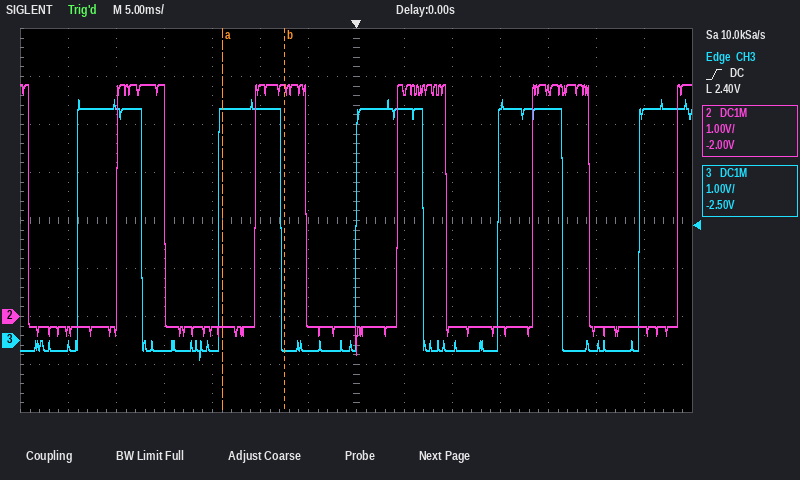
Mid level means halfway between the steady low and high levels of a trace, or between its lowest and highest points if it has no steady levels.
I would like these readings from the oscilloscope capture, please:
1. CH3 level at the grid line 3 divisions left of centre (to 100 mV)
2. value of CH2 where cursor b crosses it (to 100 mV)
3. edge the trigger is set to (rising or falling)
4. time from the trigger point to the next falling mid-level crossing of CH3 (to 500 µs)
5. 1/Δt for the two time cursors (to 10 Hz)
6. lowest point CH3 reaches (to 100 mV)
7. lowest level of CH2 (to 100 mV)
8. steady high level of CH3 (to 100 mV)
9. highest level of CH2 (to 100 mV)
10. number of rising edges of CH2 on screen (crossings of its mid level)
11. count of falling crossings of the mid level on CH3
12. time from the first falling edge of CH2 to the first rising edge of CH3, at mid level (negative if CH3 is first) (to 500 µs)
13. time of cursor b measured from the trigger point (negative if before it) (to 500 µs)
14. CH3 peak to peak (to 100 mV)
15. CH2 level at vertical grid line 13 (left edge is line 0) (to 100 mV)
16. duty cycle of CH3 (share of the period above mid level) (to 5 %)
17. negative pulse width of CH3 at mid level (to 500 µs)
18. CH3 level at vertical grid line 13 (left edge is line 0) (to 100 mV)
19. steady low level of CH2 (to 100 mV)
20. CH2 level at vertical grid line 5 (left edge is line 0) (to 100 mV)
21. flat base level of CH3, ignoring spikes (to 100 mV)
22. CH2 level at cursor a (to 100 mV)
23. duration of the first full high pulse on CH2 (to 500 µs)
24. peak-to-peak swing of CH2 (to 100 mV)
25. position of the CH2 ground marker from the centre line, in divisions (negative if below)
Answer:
-200 mV
4.7 V
rising
7.0 ms
150 Hz
-400 mV
-800 mV
4.8 V
4.8 V
5
4
+5.0 ms
-7.5 ms
5.4 V
-200 mV
45 %
8.0 ms
4.8 V
-200 mV
4.8 V
-200 mV
-200 mV
5.0 ms
5.6 V
-2.0 div
